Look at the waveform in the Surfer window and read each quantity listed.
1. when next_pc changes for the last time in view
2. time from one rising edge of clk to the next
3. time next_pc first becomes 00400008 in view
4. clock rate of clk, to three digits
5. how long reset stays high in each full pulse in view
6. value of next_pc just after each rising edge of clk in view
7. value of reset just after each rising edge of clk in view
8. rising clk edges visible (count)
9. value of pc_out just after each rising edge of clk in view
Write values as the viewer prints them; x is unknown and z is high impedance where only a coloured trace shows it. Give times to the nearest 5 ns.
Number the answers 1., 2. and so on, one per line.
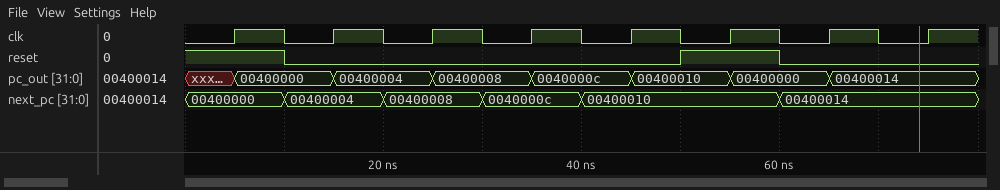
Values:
1. 60 ns
2. 10 ns
3. 20 ns
4. 100 MHz
5. 10 ns
6. 00400000, 00400004, 00400008, 0040000c, 00400010, 00400010, 00400014, 00400014
7. 1 0 0 0 0 1 0 0
8. 8
9. 00400000, 00400004, 00400008, 0040000c, 00400010, 00400000, 00400014, 00400014
